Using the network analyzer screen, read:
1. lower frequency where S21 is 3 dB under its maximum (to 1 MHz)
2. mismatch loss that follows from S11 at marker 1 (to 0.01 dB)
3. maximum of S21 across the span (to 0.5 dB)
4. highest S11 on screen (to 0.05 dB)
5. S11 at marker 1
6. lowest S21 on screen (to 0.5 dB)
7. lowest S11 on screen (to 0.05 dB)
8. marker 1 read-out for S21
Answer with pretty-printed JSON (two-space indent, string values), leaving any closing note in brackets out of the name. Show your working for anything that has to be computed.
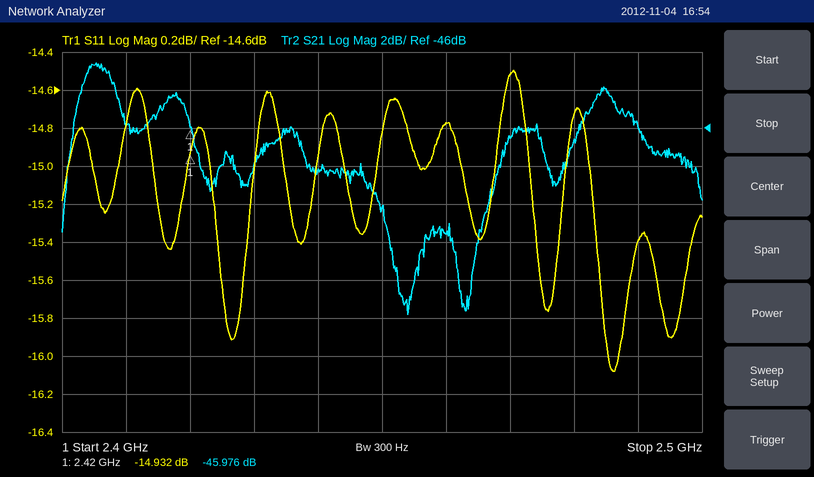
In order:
{
  "lower frequency where S21 is 3 dB under its maximum": "2.402 GHz",
  "mismatch loss that follows from S11 at marker 1": "−10 log10(1 − 10^(-14.932/10)) ≈ 0.14 dB",
  "maximum of S21 across the span": "-42.5 dB",
  "highest S11 on screen": "-14.50 dB",
  "S11 at marker 1": "-14.932 dB",
  "lowest S21 on screen": "-56.0 dB",
  "lowest S11 on screen": "-16.10 dB",
  "marker 1 read-out for S21": "-45.976 dB"
}
